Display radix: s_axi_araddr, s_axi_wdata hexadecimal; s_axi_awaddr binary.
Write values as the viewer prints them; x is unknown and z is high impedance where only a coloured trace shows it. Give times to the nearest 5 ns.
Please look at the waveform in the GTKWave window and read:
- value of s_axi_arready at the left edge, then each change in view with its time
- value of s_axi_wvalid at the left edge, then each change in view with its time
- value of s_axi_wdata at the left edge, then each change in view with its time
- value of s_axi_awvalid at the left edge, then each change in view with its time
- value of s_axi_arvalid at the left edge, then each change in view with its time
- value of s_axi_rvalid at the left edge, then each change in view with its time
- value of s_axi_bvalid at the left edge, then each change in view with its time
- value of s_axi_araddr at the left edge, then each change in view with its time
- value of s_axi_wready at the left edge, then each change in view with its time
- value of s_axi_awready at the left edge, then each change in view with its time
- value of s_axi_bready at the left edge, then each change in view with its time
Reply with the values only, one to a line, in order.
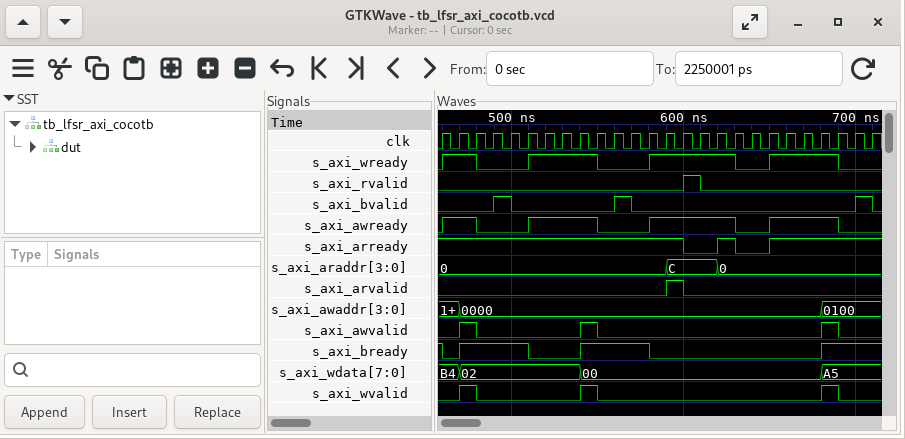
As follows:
1, 0 at 600 ns, 1 at 620 ns, 0 at 630 ns, 1 at 650 ns
0, 1 at 470 ns, 0 at 480 ns, 1 at 540 ns, 0 at 550 ns, 1 at 680 ns, 0 at 690 ns
B4, 02 at 470 ns, 00 at 540 ns, A5 at 680 ns
0, 1 at 470 ns, 0 at 480 ns, 1 at 540 ns, 0 at 550 ns, 1 at 680 ns, 0 at 690 ns
0, 1 at 590 ns, 0 at 600 ns
0, 1 at 600 ns, 0 at 610 ns
0, 1 at 490 ns, 0 at 500 ns, 1 at 560 ns, 0 at 570 ns, 1 at 700 ns, 0 at 710 ns
0, C at 590 ns, 0 at 620 ns
0, 1 at 460 ns, 0 at 480 ns, 1 at 510 ns, 0 at 550 ns, 1 at 580 ns, 0 at 630 ns, 1 at 650 ns, 0 at 690 ns
0, 1 at 460 ns, 0 at 480 ns, 1 at 510 ns, 0 at 550 ns, 1 at 580 ns, 0 at 630 ns, 1 at 650 ns, 0 at 690 ns
1, 0 at 460 ns, 1 at 470 ns, 0 at 510 ns, 1 at 540 ns, 0 at 580 ns, 1 at 680 ns
